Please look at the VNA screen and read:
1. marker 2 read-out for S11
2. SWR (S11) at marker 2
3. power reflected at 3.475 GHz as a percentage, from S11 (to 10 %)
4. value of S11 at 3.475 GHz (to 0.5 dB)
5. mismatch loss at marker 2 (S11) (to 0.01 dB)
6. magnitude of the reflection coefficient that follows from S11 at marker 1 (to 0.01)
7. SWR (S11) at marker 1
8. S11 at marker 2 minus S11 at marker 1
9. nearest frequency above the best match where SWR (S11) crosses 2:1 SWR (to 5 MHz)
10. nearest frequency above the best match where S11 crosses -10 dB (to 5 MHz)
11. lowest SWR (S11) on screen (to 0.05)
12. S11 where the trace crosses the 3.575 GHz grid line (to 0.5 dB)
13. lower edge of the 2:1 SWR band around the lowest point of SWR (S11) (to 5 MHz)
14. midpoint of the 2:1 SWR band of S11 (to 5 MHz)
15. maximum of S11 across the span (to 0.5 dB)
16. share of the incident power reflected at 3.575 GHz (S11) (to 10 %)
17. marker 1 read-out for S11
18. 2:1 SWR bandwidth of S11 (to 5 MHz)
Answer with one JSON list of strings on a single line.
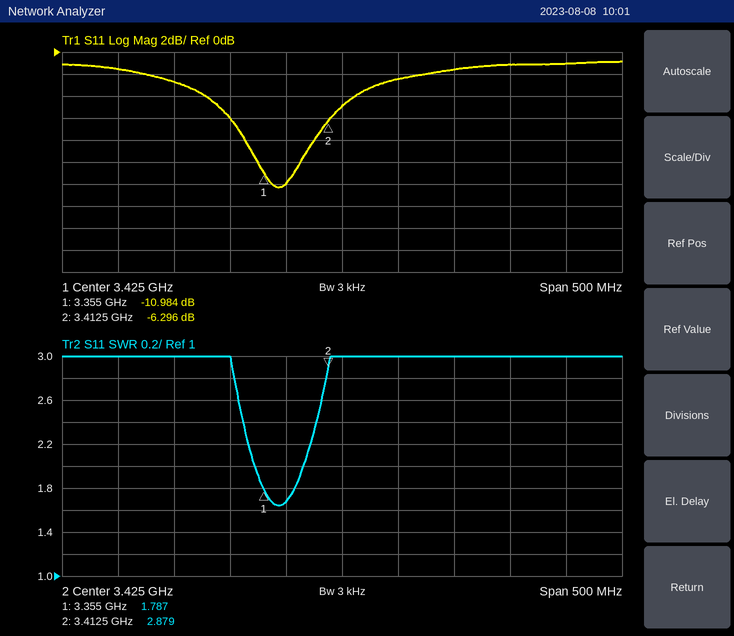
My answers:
["-6.296 dB", "2.879", "60 %", "-2.5 dB", "1.16 dB", "0.28", "1.787", "4.688 dB", "3.390 GHz", "3.390 GHz", "1.65", "-1.0 dB", "3.345 GHz", "3.370 GHz", "-1.0 dB", "80 %", "-10.984 dB", "45 MHz"]
